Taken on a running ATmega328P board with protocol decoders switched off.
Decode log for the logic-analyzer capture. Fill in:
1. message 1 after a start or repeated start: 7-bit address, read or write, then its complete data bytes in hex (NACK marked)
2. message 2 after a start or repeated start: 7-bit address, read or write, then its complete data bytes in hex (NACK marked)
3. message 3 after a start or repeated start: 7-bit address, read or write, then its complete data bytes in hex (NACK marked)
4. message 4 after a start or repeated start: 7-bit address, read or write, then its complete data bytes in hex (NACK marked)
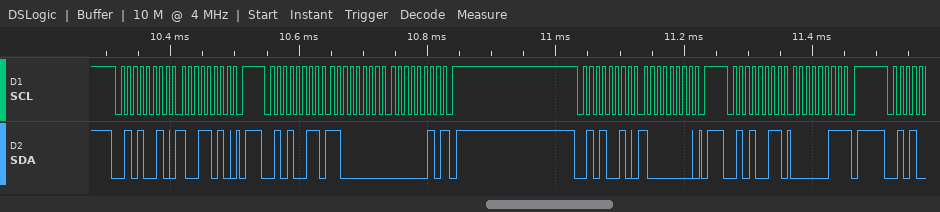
0x29 write: 9A
0x29 read: C0 02 NACK
0x29 write: 80
0x29 read: 03 NACK
